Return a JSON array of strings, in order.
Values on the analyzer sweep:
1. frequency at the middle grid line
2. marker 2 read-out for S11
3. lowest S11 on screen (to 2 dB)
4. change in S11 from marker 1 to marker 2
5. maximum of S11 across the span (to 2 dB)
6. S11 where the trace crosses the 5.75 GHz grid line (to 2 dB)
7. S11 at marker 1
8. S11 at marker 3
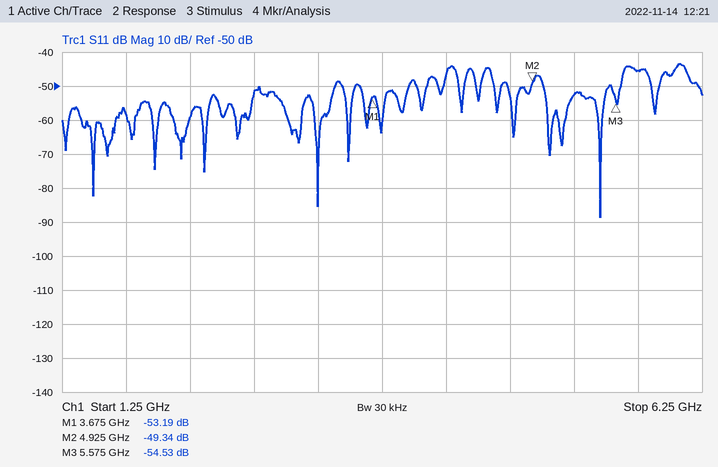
["3.75 GHz", "-49.34 dB", "-88 dB", "3.85 dB", "-44 dB", "-46 dB", "-53.19 dB", "-54.53 dB"]
